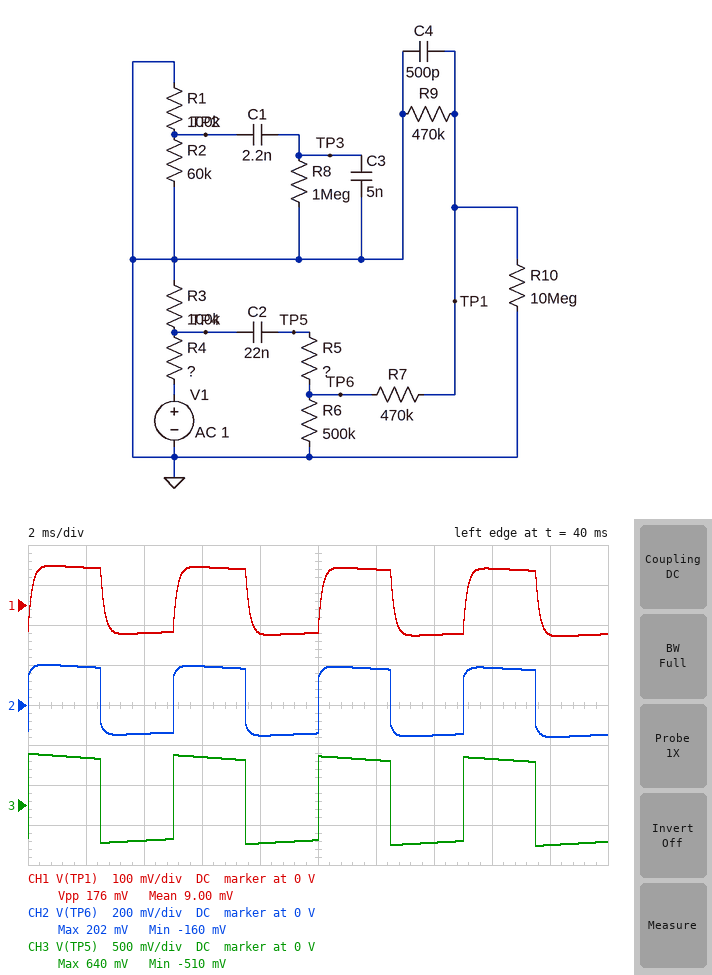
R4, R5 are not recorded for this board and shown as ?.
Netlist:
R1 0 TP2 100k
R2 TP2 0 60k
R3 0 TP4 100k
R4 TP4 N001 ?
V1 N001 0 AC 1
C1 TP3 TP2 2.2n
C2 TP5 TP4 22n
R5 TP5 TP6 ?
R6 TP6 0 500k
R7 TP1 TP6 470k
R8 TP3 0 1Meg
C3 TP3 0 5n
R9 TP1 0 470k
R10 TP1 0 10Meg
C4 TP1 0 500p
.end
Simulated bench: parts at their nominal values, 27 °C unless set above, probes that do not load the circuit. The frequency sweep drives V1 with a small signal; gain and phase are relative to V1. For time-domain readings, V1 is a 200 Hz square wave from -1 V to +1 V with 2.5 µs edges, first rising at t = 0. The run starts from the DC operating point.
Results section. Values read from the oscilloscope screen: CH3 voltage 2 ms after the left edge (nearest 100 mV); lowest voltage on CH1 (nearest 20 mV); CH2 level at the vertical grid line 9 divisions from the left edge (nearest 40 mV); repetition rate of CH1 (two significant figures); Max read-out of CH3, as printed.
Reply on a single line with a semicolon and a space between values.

600 mV; -80 mV; -160 mV; 200 Hz; 640 mV
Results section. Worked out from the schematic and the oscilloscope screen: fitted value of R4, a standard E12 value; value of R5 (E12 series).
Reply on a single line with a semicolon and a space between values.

82 kΩ; 680 kΩ
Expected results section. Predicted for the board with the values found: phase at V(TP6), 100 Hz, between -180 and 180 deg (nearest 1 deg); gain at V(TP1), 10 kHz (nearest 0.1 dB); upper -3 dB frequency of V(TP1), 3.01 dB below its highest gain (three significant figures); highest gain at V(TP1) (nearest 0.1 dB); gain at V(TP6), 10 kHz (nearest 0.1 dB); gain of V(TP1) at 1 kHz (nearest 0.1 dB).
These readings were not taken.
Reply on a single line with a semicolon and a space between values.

3 deg; -40.7 dB; 1.14 kHz; -21.7 dB; -17.2 dB; -24.2 dB
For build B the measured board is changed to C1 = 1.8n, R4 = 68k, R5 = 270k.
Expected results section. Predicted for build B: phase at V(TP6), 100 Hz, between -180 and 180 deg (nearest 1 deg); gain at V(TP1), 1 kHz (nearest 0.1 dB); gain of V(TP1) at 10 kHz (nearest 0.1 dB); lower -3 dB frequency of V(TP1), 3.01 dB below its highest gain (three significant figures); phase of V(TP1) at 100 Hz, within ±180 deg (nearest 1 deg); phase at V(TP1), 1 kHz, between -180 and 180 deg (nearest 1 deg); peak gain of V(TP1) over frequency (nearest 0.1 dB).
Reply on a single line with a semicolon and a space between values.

6 deg; -18.9 dB; -35.1 dB; 11.2 Hz; 2 deg; -39 deg; -16.7 dB
